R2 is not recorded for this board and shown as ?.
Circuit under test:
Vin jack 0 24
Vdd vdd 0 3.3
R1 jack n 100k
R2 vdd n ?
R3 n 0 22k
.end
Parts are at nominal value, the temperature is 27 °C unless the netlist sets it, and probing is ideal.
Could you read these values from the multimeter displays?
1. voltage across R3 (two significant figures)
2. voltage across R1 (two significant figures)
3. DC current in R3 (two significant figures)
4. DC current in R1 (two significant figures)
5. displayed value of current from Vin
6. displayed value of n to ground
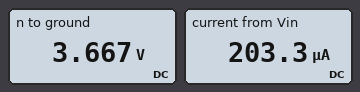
3.7 V
20 V
170 µA
200 µA
203.3 µA
3.667 V
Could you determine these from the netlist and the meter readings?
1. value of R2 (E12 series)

10 kΩ
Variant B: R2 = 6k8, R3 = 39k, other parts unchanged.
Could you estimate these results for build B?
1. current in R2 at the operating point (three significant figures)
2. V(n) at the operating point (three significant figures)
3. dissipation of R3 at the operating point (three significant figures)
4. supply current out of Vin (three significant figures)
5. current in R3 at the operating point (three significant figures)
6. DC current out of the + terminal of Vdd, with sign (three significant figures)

98.5 µA
3.97 V
404 µW
200 µA
102 µA
-98.5 µA
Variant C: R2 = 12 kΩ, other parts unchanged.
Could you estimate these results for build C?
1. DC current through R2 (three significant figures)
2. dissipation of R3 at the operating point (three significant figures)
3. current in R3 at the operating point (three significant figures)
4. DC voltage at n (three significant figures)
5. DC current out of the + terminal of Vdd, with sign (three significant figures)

34.2 µA
626 µW
169 µA
3.71 V
-34.2 µA
